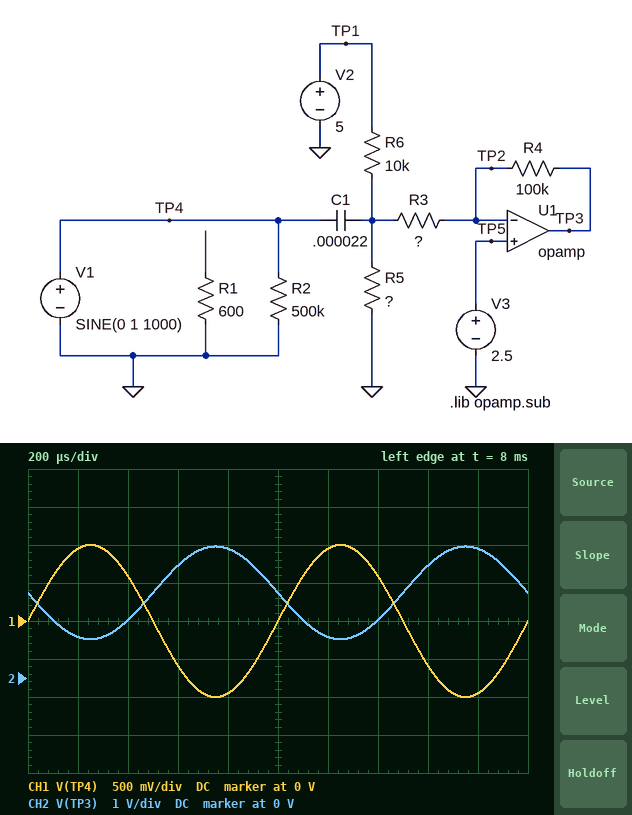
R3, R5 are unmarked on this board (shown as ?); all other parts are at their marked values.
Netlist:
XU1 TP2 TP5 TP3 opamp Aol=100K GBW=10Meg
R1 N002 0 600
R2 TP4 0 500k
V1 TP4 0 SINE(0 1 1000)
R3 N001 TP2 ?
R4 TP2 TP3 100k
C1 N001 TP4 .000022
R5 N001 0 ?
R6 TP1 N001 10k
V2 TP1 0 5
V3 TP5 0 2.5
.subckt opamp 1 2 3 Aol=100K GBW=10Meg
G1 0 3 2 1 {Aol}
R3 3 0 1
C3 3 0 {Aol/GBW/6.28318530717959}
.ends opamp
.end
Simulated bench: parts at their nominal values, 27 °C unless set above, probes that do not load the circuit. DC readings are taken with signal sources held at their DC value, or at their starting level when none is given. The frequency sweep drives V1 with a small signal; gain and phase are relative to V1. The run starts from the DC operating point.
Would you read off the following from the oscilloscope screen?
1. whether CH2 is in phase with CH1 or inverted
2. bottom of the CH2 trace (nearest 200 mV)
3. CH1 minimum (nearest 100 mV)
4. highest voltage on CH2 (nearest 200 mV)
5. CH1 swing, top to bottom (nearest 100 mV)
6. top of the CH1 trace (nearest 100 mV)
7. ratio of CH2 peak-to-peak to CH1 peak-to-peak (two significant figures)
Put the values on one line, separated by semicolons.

inverted; 1.0 V; -1.0 V; 3.4 V; 2.0 V; 1.0 V; 1.2
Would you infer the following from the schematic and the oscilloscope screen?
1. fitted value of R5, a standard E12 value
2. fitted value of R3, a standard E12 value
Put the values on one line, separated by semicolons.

12 kΩ; 82 kΩ
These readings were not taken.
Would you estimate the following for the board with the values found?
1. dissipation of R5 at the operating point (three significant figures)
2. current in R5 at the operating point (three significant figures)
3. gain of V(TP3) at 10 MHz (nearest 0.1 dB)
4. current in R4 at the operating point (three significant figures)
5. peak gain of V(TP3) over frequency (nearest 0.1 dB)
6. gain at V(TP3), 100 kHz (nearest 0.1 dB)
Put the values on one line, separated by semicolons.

613 µW; 226 µA; -6.0 dB; 2.60 µA; 1.7 dB; 1.7 dB
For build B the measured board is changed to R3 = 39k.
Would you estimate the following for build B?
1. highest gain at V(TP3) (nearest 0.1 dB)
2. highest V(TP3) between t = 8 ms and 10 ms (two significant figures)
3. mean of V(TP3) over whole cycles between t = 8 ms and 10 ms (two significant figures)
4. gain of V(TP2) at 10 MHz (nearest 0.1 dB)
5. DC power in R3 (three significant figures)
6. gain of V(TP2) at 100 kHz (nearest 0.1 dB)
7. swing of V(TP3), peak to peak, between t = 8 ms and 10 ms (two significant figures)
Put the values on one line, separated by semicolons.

8.2 dB; 4.6 V; 2.0 V; -3.2 dB; 1.02 µW; -31.8 dB; 5.1 V
